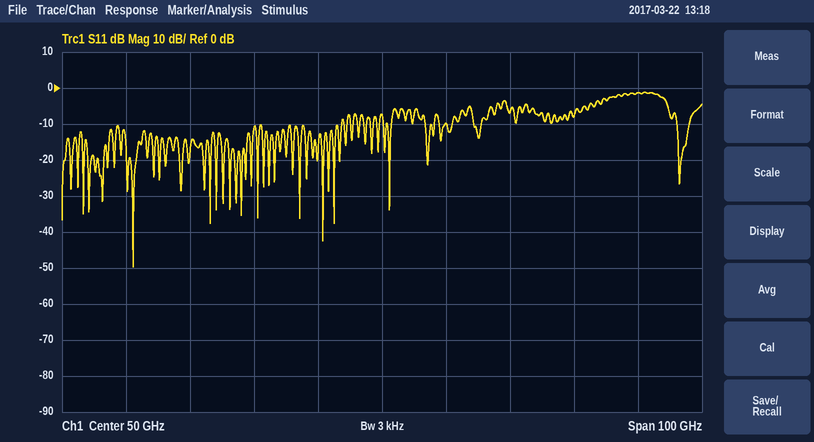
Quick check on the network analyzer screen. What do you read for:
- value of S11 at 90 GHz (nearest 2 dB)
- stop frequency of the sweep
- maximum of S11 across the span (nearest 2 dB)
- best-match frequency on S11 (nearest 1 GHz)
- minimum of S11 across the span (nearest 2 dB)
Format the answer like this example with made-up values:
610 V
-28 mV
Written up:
-2 dB
100 GHz
-2 dB
11 GHz
-50 dB
